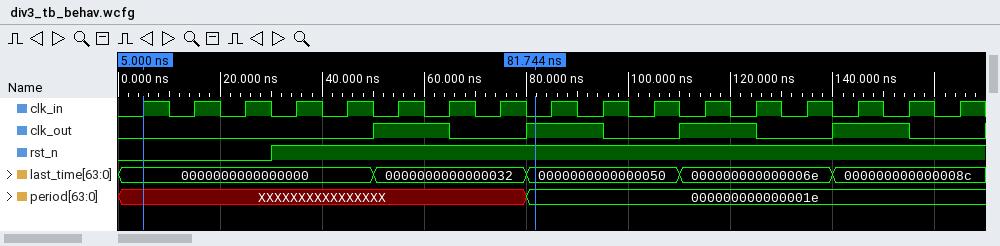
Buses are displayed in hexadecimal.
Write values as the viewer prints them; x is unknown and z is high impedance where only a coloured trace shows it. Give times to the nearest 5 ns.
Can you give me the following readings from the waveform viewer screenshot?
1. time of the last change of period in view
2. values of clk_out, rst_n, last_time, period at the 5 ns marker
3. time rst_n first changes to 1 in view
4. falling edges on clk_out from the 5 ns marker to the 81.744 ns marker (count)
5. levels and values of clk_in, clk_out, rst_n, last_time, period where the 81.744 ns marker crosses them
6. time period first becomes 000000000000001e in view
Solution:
80 ns
clk_out=0, rst_n=0, last_time=0000000000000000, period=XXXXXXXXXXXXXXXX
30 ns
1
clk_in=0, clk_out=1, rst_n=1, last_time=0000000000000050, period=000000000000001e
80 ns
